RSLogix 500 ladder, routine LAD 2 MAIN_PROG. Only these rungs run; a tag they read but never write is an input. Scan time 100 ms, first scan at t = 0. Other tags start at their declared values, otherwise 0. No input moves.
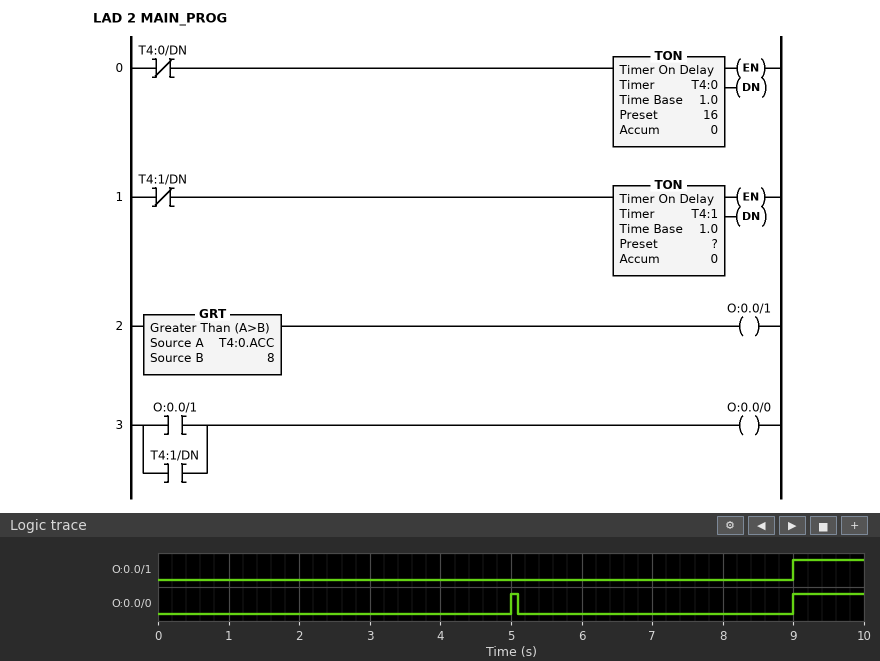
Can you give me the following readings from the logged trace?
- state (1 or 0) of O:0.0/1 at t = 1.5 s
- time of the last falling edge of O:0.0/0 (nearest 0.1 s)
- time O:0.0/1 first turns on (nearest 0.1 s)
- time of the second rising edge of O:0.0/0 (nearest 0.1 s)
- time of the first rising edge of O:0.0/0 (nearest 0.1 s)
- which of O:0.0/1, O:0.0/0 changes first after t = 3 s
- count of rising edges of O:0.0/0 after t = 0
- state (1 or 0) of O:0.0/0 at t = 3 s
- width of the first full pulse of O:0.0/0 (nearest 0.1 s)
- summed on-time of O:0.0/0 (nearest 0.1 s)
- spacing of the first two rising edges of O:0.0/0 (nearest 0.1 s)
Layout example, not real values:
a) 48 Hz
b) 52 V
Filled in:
a) 0
b) 5.1 s
c) 9.0 s
d) 9.0 s
e) 5.0 s
f) O:0.0/0
g) 2
h) 0
i) 0.1 s
j) 1.1 s
k) 4.0 s
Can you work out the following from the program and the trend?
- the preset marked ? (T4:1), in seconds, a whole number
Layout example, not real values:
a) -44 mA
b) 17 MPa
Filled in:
a) 5 s
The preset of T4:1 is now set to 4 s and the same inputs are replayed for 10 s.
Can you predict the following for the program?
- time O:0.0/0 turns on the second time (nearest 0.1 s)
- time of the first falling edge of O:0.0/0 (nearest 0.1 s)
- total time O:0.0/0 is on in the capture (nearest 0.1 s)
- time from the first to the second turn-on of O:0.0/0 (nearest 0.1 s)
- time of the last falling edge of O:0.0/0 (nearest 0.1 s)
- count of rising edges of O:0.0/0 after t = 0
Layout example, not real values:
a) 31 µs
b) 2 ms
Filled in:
a) 8.2 s
b) 4.1 s
c) 1.2 s
d) 4.2 s
e) 8.3 s
f) 3
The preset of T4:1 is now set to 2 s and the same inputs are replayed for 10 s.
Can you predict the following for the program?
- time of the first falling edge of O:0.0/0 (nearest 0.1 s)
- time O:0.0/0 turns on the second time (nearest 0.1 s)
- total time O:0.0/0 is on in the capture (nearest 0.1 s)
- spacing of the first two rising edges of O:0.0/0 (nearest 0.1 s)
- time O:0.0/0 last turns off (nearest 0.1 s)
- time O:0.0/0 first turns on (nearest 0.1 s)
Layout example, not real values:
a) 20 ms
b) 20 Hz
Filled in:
a) 2.1 s
b) 4.2 s
c) 1.4 s
d) 2.2 s
e) 8.7 s
f) 2.0 s
